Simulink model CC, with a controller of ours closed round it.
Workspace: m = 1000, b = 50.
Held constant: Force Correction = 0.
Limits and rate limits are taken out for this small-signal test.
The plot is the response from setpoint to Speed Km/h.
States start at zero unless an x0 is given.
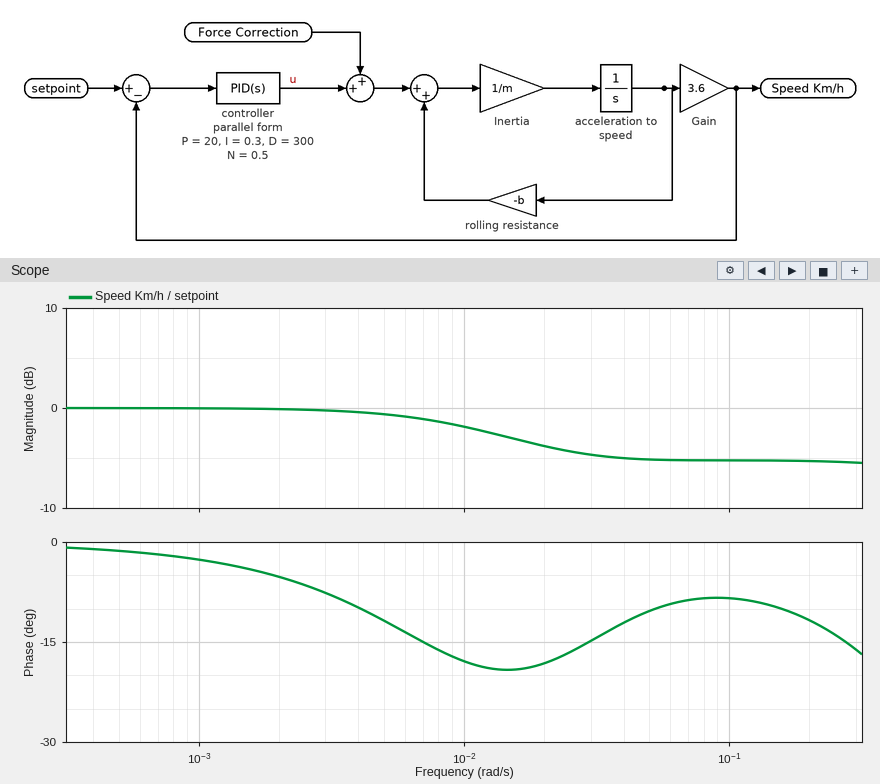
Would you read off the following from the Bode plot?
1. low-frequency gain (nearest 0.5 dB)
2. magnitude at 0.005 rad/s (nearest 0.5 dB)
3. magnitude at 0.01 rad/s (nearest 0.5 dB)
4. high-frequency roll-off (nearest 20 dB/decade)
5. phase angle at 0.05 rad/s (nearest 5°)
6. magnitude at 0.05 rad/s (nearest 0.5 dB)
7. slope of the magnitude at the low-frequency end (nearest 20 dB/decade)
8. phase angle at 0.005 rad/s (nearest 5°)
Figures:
0.0 dB
-0.5 dB
-2.0 dB
0 dB/decade
-10°
-5.0 dB
0 dB/decade
-10°
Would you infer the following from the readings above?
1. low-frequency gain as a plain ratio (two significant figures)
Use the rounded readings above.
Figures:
1.0
